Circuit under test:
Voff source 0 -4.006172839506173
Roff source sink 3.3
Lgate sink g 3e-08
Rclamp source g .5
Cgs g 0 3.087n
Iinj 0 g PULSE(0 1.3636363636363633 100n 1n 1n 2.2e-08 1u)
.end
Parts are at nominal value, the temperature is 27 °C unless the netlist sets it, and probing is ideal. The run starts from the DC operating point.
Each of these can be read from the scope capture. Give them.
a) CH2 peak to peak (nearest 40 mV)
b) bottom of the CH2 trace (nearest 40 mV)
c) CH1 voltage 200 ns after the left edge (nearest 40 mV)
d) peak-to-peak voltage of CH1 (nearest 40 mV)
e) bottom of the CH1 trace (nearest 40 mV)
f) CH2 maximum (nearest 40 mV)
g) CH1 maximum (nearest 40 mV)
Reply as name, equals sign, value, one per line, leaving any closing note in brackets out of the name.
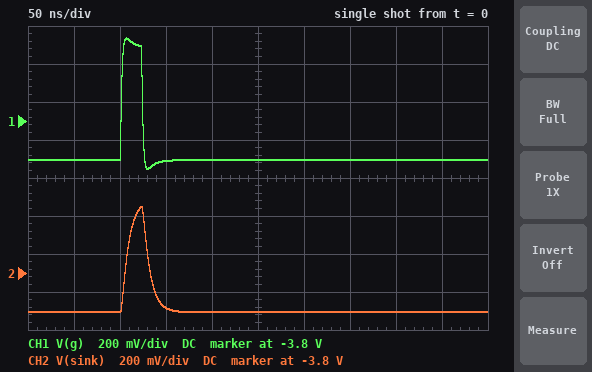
CH2 peak to peak = 560 mV
bottom of the CH2 trace = -4.00 V
CH1 voltage 200 ns after the left edge = -4.00 V
peak-to-peak voltage of CH1 = 680 mV
bottom of the CH1 trace = -4.04 V
CH2 maximum = -3.44 V
CH1 maximum = -3.36 V
